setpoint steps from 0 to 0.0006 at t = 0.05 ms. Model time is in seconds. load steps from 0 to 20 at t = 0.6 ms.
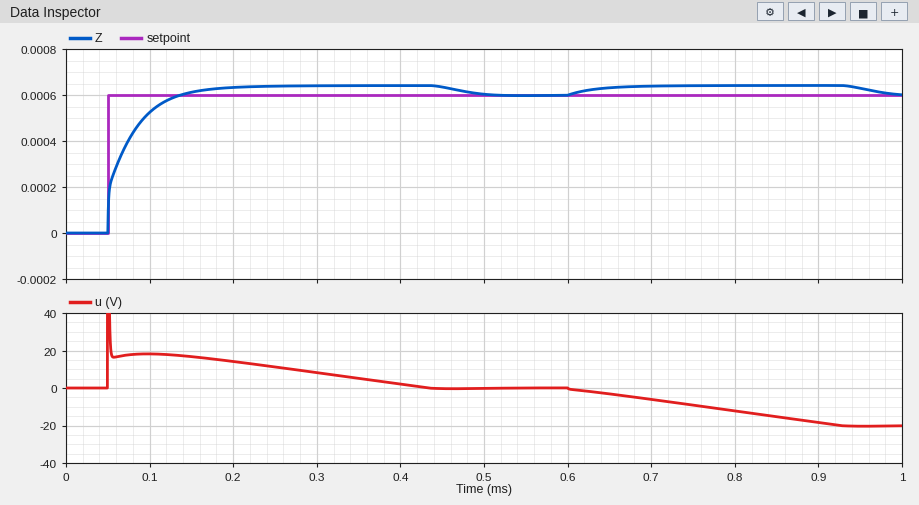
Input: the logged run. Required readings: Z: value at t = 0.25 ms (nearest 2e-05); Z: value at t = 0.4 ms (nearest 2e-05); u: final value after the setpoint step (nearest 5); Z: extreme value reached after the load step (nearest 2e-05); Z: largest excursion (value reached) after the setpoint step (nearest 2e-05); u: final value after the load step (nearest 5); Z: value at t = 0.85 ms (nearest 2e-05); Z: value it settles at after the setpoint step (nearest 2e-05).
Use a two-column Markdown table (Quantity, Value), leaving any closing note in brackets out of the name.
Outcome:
| Quantity | Value |
|---|---|
| Z: value at t = 0.25 ms | 0.00064 |
| Z: value at t = 0.4 ms | 0.00064 |
| u: final value after the setpoint step | 0 |
| Z: extreme value reached after the load step | 0.00064 |
| Z: largest excursion (value reached) after the setpoint step | 0.00064 |
| u: final value after the load step | -20 |
| Z: value at t = 0.85 ms | 0.00064 |
| Z: value it settles at after the setpoint step | 0.00060 |
